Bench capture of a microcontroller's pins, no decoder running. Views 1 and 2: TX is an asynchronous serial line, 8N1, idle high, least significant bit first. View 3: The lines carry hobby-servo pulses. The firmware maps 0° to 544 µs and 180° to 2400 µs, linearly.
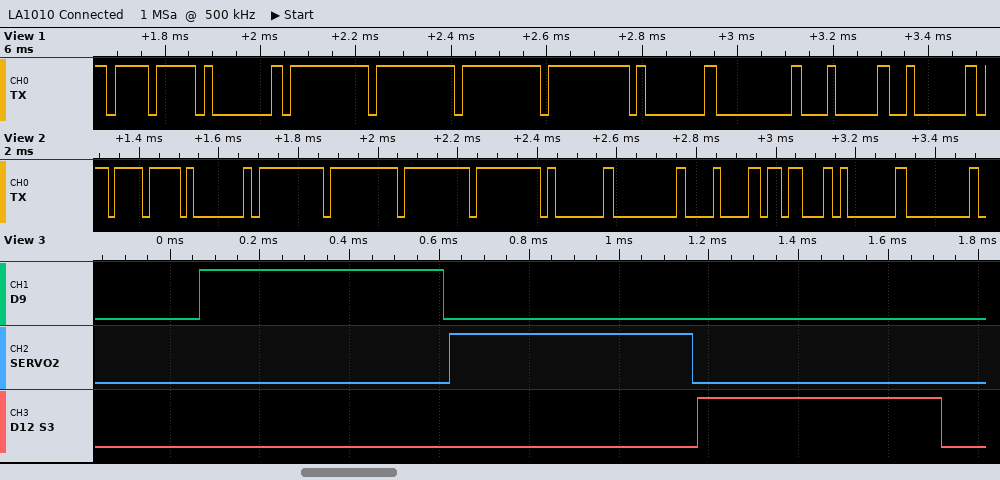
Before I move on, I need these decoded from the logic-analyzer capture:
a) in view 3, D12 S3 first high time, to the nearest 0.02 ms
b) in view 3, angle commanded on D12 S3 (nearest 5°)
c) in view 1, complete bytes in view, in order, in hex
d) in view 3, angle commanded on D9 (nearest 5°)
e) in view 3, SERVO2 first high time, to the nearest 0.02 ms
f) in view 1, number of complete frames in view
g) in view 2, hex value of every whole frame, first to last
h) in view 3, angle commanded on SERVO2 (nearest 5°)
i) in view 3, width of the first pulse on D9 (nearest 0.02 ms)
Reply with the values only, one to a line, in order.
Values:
0.54 ms
0°
EF 01 FF FF FF FF 01 00 04 02
0°
0.54 ms
10
0xEF 0x01 0xFF 0xFF 0xFF 0xFF 0x01 0x00 0x08 0x1B 0x01 0x00
0°
0.54 ms
